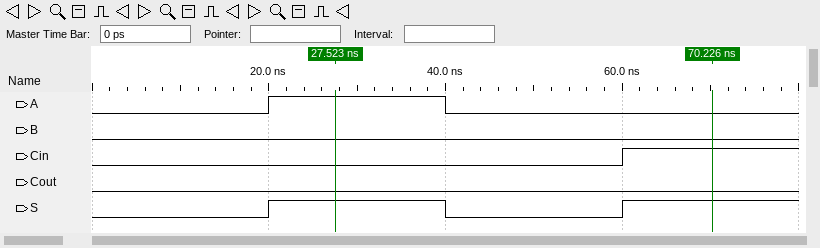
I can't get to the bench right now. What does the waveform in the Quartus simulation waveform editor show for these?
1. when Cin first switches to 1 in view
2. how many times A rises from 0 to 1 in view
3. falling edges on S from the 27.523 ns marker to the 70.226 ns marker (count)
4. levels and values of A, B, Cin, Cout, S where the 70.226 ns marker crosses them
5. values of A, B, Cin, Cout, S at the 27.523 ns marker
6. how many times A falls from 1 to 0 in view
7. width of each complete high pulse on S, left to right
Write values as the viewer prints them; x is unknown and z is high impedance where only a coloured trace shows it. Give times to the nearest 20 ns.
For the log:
60 ns
1
1
A=0, B=0, Cin=1, Cout=0, S=1
A=1, B=0, Cin=0, Cout=0, S=1
1
20 ns
